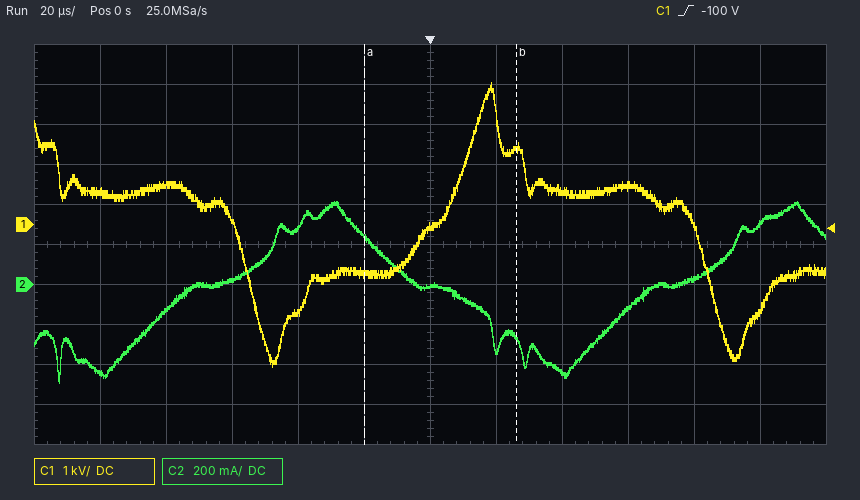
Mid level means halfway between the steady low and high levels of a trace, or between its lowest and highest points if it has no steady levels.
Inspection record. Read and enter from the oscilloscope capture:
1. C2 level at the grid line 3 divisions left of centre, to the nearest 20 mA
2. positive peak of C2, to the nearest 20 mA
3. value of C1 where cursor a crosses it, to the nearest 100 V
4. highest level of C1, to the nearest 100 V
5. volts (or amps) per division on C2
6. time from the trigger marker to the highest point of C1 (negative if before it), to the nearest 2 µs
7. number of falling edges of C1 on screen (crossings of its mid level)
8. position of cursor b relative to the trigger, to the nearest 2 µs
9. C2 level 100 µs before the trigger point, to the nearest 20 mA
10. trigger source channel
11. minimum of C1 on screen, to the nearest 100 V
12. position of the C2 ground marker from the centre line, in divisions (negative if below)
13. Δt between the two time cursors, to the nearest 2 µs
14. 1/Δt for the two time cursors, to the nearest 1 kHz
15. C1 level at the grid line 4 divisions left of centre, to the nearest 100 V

20 mA
420 mA
-1.2 kV
3.6 kV
200 mA
+18 µs
2
+26 µs
-440 mA
C1
-3.6 kV
-1.0 div
46 µs
22 kHz
1.0 kV
